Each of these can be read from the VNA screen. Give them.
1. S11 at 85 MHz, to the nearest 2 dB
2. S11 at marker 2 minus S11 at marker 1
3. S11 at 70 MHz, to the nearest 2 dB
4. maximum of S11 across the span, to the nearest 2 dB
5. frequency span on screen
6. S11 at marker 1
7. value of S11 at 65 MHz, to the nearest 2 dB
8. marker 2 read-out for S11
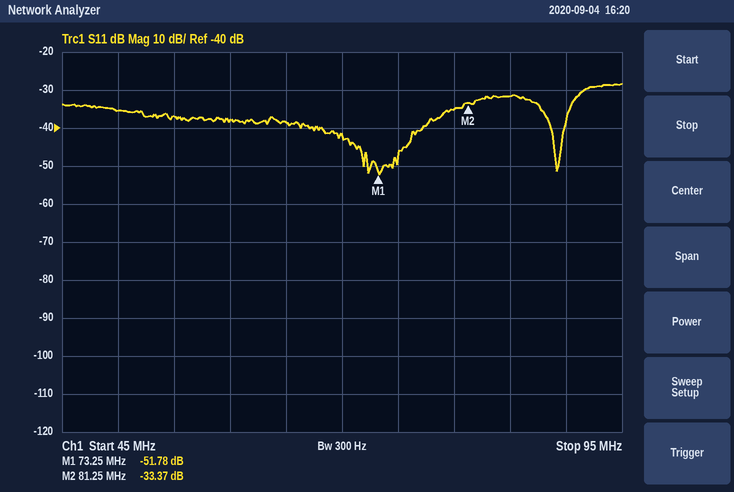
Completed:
-32 dB
18.41 dB
-42 dB
-28 dB
50 MHz
-51.78 dB
-38 dB
-33.37 dB
